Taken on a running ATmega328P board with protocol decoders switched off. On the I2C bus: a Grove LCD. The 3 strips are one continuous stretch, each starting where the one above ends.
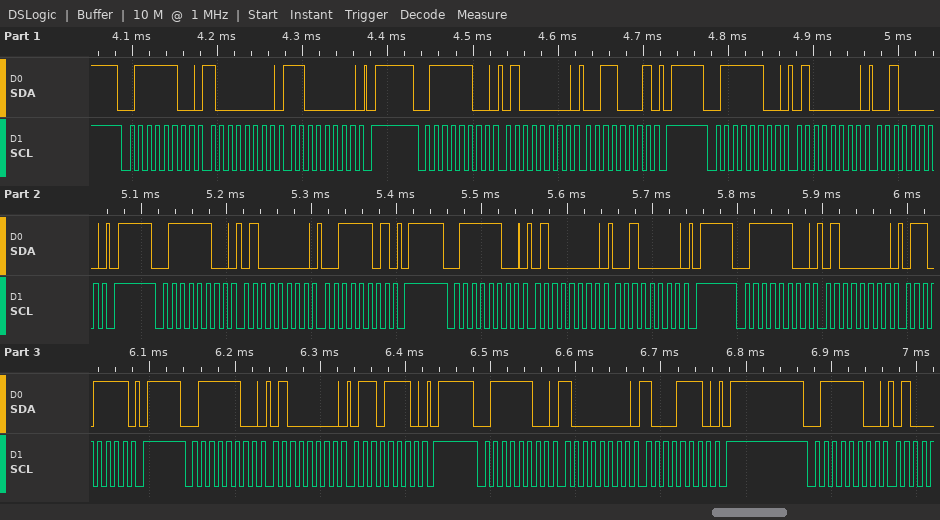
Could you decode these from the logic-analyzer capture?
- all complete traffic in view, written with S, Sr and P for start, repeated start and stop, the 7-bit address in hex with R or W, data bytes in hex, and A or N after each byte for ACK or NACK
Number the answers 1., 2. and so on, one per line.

1. S 3EW A 80 A C0 A P S 3EW A 40 A 31 A P S 3EW A 40 A 20 A P S 3EW A 40 A 3D A P S 3EW A 40 A 20 A P S 3EW A 40 A 6F A P S 3EW A 40 A 6E A P S 3EW A 80 A 8E A P S 3EW A
